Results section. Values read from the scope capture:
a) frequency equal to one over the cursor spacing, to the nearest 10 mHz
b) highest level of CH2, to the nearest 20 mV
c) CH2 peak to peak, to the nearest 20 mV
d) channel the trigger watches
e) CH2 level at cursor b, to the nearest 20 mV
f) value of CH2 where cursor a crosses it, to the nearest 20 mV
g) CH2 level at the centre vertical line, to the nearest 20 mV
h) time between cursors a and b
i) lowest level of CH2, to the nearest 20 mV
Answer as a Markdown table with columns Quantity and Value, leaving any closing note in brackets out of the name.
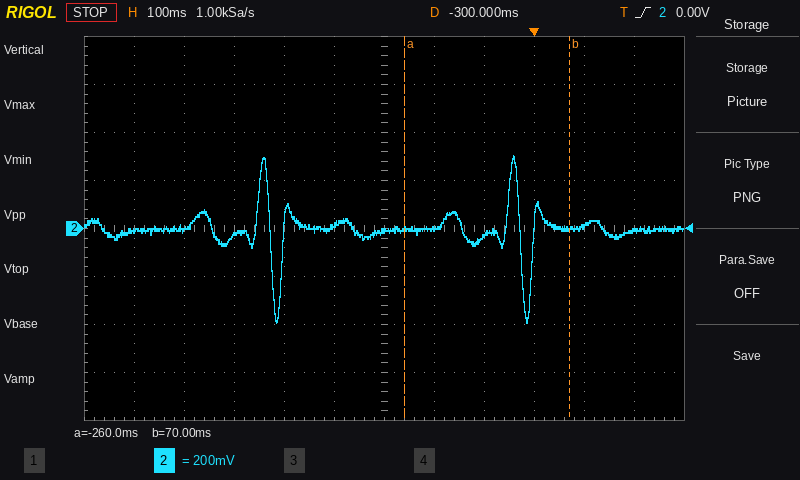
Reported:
| Quantity | Value |
|---|---|
| frequency equal to one over the cursor spacing, to the nearest 10 mHz | 3.03 Hz |
| highest level of CH2, to the nearest 20 mV | 300 mV |
| CH2 peak to peak, to the nearest 20 mV | 700 mV |
| channel the trigger watches | CH2 |
| CH2 level at cursor b, to the nearest 20 mV | 0 mV |
| value of CH2 where cursor a crosses it, to the nearest 20 mV | 0 mV |
| CH2 level at the centre vertical line, to the nearest 20 mV | 0 mV |
| time between cursors a and b | 330 ms |
| lowest level of CH2, to the nearest 20 mV | -400 mV |
